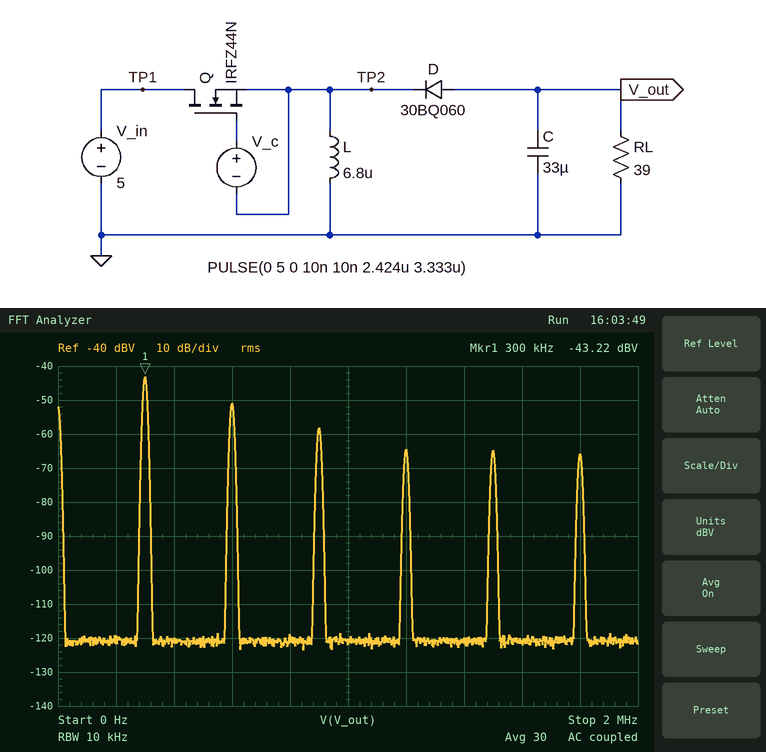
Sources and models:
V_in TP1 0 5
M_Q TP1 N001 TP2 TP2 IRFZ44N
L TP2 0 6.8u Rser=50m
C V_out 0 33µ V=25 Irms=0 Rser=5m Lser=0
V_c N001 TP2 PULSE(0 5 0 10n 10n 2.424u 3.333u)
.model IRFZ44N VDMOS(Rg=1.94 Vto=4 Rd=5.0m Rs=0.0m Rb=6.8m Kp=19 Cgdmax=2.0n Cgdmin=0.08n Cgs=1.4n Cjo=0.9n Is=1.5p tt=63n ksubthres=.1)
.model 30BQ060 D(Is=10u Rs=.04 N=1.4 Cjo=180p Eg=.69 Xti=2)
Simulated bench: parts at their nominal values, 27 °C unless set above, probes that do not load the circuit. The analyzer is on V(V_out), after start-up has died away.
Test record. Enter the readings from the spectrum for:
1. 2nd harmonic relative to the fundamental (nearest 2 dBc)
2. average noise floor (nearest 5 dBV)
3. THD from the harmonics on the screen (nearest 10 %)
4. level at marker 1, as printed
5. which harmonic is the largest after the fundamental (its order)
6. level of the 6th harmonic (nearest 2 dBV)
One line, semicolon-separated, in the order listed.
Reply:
-8 dBc; -120 dBV; 50 %; -43.22 dBV; 2; -66 dBV
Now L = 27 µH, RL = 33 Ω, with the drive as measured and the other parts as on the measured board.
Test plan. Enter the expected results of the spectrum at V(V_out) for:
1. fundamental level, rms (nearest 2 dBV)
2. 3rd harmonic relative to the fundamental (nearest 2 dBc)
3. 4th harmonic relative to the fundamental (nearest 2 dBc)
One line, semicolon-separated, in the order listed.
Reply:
-42 dBV; -18 dBc; -30 dBc
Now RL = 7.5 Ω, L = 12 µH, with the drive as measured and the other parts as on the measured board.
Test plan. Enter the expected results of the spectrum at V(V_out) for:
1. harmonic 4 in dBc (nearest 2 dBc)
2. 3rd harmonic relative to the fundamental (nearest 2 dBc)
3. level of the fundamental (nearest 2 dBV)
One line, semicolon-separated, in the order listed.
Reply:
-30 dBc; -20 dBc; -30 dBV
